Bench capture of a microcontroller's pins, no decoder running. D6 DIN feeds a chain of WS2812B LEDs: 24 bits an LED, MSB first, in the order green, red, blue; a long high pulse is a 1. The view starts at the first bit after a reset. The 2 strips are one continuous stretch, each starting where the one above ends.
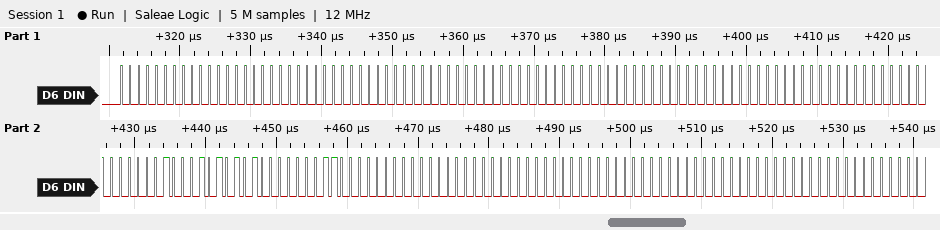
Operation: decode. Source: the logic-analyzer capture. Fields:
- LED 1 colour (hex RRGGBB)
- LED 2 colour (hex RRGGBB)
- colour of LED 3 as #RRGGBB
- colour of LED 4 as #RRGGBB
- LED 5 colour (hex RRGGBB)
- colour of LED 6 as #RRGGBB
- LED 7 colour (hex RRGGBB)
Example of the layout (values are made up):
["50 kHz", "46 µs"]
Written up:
["#000000", "#000000", "#000000", "#000000", "#A8220C", "#000000", "#000000"]
